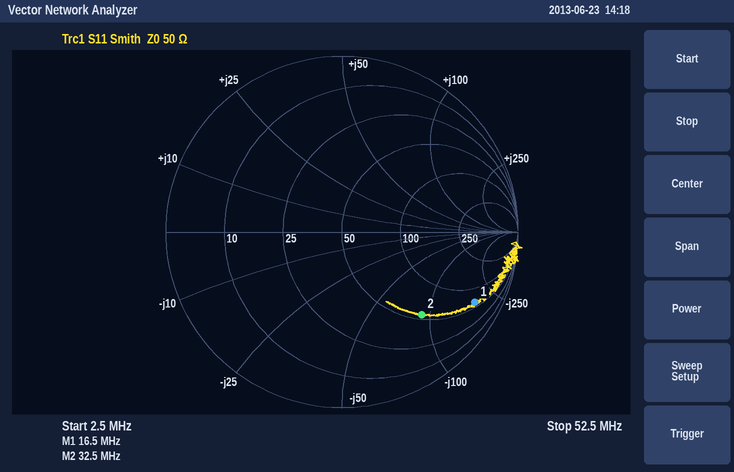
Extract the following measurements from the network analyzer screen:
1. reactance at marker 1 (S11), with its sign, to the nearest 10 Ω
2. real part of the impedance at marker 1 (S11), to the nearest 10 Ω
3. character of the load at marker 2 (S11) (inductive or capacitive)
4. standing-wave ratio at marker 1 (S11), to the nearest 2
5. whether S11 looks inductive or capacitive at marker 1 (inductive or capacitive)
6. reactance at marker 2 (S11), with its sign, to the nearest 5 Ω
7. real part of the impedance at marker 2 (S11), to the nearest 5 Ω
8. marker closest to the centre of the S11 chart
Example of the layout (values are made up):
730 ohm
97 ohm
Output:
-180 Ω
60 Ω
capacitive
12
capacitive
-90 Ω
55 Ω
marker 2
